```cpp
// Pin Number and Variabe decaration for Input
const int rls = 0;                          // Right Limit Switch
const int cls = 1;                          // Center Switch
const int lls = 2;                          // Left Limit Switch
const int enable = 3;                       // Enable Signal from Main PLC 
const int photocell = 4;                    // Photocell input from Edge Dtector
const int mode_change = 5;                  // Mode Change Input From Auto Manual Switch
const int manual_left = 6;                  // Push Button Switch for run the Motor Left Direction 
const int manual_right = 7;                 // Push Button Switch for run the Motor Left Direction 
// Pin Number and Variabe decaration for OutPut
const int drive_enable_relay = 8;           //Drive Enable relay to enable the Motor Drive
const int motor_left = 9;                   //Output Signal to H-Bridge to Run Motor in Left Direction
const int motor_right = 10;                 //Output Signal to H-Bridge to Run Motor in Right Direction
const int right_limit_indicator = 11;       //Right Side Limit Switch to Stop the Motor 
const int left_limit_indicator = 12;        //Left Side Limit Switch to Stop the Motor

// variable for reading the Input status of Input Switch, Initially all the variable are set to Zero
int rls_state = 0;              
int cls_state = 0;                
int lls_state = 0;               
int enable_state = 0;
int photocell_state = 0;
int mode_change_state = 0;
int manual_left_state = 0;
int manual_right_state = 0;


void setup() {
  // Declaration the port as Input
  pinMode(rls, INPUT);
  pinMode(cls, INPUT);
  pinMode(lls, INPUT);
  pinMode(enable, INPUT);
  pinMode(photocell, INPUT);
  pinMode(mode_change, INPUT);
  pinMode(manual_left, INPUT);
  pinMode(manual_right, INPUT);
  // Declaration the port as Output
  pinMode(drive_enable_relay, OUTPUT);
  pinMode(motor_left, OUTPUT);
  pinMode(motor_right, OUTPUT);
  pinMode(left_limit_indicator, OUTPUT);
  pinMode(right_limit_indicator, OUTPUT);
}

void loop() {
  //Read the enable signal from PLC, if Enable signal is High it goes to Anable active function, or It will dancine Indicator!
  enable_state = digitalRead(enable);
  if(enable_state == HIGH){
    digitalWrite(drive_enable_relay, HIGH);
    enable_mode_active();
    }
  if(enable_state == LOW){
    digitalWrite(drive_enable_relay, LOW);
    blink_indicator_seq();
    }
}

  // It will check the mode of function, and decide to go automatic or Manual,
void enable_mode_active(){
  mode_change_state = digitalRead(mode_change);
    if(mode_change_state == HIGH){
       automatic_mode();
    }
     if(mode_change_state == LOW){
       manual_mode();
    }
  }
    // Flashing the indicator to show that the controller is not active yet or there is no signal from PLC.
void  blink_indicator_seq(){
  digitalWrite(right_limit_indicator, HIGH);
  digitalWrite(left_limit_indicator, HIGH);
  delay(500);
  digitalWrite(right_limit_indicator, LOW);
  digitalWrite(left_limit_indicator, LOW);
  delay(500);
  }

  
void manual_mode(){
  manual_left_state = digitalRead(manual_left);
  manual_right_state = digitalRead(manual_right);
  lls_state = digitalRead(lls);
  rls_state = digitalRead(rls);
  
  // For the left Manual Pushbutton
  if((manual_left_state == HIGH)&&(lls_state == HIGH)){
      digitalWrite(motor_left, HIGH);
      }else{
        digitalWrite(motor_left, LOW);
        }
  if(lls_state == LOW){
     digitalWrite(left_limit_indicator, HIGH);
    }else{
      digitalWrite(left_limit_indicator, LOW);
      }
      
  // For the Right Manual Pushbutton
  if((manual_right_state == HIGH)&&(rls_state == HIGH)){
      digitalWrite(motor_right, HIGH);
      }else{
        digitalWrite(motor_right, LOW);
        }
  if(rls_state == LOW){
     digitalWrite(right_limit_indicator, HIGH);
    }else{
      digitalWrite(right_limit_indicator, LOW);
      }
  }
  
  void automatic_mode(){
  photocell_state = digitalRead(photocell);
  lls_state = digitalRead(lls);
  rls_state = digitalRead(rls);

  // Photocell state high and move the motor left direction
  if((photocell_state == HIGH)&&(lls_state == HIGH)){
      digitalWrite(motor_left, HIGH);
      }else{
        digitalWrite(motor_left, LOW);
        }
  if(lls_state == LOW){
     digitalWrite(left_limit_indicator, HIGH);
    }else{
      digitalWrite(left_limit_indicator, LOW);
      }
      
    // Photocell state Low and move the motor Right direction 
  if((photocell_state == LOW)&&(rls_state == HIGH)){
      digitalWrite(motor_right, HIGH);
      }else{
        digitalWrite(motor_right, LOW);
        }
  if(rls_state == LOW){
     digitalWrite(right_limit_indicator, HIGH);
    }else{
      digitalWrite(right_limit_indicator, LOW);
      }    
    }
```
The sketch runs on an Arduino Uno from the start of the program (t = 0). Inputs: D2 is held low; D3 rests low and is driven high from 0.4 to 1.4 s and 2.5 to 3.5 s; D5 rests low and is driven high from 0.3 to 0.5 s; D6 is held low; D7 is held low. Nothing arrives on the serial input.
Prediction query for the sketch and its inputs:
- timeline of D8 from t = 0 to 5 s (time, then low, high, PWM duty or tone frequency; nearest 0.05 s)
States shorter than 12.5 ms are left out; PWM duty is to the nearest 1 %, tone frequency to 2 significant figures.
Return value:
0 s low; 1 s high; 1.4 s low; 3.4 s high; 3.5 s low
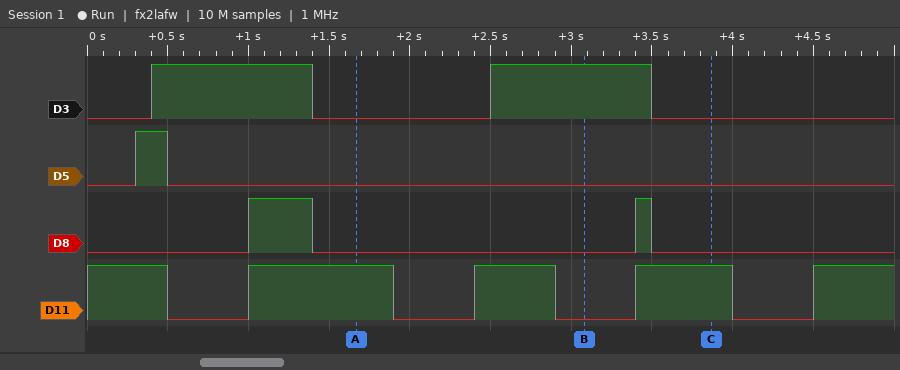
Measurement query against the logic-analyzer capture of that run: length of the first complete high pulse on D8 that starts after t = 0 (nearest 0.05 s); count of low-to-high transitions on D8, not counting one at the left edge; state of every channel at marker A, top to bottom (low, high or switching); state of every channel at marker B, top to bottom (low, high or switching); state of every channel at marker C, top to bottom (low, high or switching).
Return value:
0.40 s
2
D3 low, D5 low, D8 low, D11 high
D3 high, D5 low, D8 low, D11 low
D3 low, D5 low, D8 low, D11 high
